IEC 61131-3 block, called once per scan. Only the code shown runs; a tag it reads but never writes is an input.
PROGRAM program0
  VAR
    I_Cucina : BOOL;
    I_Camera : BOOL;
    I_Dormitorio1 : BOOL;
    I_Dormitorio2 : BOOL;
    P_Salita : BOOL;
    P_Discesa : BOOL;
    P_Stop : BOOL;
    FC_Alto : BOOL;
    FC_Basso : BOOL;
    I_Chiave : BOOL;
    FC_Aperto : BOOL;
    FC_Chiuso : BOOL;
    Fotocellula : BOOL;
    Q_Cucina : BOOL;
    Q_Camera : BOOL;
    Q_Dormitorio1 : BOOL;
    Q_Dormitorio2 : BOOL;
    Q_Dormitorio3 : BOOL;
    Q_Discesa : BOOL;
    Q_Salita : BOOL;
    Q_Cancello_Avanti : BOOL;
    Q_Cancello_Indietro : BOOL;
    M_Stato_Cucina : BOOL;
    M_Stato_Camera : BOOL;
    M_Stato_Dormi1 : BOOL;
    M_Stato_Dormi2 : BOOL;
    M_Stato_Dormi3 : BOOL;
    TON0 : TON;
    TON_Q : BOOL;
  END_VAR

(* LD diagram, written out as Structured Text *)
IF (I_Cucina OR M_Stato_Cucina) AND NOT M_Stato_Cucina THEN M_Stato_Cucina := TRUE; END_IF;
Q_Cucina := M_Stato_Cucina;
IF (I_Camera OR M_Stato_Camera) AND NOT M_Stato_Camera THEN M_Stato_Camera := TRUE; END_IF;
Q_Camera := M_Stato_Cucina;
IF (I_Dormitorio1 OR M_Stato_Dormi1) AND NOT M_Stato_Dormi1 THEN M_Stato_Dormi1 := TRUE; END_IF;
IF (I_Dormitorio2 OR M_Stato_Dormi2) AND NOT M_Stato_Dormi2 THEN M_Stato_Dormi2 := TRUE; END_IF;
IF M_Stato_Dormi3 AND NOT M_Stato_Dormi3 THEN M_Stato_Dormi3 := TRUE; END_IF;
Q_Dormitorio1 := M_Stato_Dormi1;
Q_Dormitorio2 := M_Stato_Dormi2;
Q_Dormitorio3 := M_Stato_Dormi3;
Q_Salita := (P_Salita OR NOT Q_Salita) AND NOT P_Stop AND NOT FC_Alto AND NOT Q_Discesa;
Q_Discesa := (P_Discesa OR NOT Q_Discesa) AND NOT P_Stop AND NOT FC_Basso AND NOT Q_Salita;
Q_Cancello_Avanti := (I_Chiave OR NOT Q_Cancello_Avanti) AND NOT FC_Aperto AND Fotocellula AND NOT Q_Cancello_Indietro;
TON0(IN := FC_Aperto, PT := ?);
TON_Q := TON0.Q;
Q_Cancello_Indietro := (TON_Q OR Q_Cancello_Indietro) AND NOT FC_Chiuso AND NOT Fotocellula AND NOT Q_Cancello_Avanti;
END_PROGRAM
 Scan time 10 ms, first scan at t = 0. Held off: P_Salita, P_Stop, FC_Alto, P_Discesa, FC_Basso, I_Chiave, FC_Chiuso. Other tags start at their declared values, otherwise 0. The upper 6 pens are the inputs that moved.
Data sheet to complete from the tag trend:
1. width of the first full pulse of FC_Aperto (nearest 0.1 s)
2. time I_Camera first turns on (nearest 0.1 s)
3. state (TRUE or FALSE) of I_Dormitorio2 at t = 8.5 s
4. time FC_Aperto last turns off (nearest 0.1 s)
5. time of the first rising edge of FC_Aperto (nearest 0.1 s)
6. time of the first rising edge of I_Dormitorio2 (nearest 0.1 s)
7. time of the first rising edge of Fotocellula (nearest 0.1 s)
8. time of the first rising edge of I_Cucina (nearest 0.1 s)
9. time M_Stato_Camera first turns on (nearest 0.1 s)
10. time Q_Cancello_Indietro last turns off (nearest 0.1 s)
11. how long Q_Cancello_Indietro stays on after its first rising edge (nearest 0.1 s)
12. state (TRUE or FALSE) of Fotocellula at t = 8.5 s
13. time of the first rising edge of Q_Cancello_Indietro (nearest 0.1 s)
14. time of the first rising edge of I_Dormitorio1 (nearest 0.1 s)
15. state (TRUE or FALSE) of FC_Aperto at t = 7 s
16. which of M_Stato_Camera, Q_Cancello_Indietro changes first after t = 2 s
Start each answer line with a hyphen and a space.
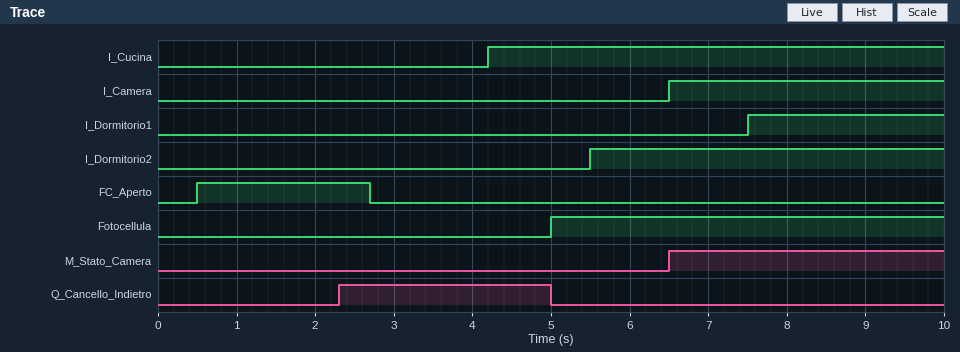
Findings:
- 2.2 s
- 6.5 s
- TRUE
- 2.7 s
- 0.5 s
- 5.5 s
- 5.0 s
- 4.2 s
- 6.5 s
- 5.0 s
- 2.7 s
- TRUE
- 2.3 s
- 7.5 s
- FALSE
- Q_Cancello_Indietro
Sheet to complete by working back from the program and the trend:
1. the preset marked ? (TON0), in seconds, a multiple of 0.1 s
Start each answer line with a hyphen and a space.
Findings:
- 1.8 s
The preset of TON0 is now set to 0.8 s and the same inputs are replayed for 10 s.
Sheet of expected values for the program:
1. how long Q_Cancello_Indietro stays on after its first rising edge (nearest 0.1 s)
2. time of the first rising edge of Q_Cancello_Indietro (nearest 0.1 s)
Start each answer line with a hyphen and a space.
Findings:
- 3.7 s
- 1.3 s
